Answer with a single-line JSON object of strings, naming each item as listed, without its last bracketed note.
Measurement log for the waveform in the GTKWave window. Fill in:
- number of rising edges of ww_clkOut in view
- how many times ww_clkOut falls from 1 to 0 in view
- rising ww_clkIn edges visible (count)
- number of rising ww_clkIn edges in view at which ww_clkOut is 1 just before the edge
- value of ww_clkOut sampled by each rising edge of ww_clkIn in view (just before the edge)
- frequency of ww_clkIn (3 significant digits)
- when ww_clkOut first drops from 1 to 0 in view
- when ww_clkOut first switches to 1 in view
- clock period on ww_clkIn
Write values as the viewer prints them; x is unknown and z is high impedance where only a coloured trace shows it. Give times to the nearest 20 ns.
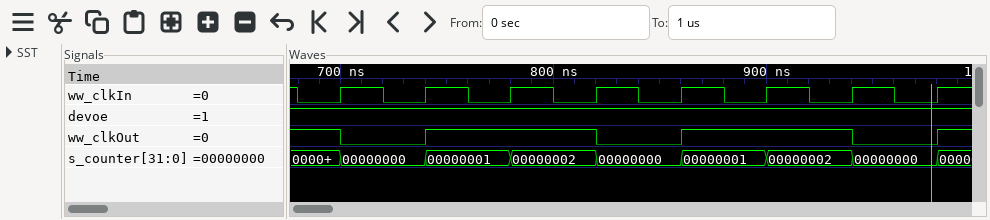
{"number of rising edges of ww_clkOut in view": "3", "how many times ww_clkOut falls from 1 to 0 in view": "3", "rising ww_clkIn edges visible": "8", "number of rising ww_clkIn edges in view at which ww_clkOut is 1 just before the edge": "5", "value of ww_clkOut sampled by each rising edge of ww_clkIn in view": "1 0 1 1 0 1 1 0", "frequency of ww_clkIn": "25.0 MHz", "when ww_clkOut first drops from 1 to 0 in view": "700 ns", "when ww_clkOut first switches to 1 in view": "740 ns", "clock period on ww_clkIn": "40 ns"}
